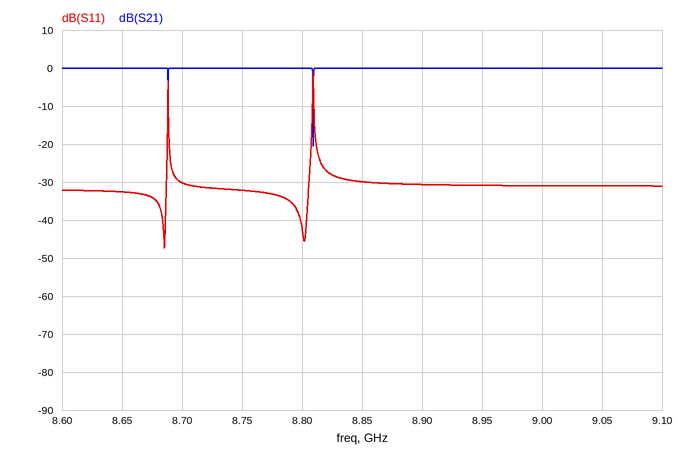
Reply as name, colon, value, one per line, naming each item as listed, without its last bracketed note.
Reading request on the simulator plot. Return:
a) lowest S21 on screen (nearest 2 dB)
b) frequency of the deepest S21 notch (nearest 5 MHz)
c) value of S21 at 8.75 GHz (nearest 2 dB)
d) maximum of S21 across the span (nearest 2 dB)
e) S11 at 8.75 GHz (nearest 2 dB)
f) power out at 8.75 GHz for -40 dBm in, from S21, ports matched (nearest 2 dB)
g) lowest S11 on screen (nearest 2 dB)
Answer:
lowest S21 on screen: -20 dB
frequency of the deepest S21 notch: 8.810 GHz
value of S21 at 8.75 GHz: 0 dB
maximum of S21 across the span: 0 dB
S11 at 8.75 GHz: -32 dB
power out at 8.75 GHz for -40 dBm in, from S21, ports matched: -40 dBm
lowest S11 on screen: -48 dB
